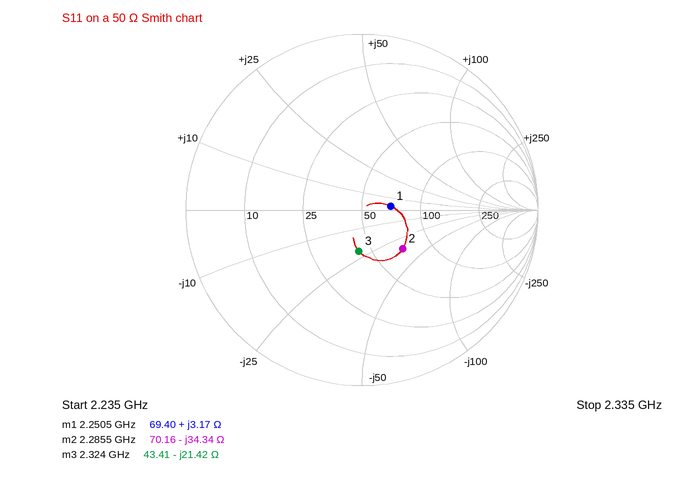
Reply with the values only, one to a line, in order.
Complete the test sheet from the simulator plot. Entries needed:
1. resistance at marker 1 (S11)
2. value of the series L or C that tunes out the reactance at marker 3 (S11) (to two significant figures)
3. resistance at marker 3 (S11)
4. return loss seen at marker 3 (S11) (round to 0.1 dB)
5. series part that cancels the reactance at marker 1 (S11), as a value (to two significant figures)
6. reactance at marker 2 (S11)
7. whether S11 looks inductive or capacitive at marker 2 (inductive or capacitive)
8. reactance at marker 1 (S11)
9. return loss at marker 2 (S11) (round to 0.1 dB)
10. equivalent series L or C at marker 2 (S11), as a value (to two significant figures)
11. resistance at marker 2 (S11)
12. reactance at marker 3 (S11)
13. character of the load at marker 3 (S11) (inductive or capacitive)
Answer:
69.40 Ω
1.5 nH
43.41 Ω
12.6 dB
22 pF
-34.34 Ω
capacitive
+3.17 Ω
9.9 dB
2.0 pF
70.16 Ω
-21.42 Ω
capacitive
